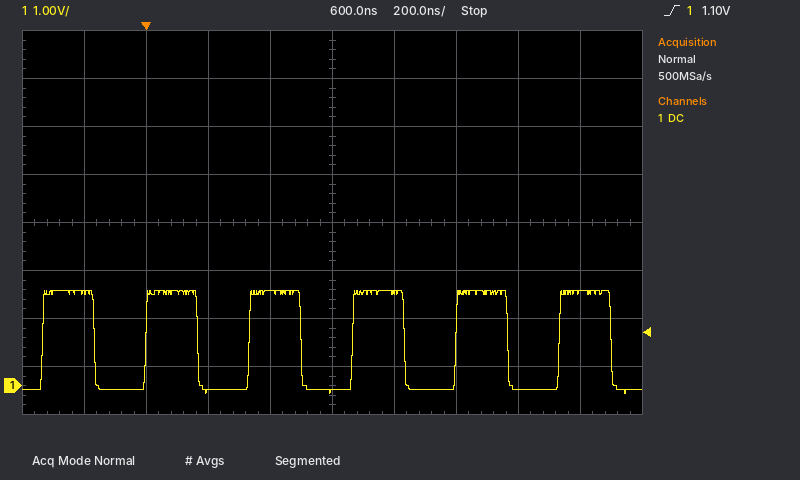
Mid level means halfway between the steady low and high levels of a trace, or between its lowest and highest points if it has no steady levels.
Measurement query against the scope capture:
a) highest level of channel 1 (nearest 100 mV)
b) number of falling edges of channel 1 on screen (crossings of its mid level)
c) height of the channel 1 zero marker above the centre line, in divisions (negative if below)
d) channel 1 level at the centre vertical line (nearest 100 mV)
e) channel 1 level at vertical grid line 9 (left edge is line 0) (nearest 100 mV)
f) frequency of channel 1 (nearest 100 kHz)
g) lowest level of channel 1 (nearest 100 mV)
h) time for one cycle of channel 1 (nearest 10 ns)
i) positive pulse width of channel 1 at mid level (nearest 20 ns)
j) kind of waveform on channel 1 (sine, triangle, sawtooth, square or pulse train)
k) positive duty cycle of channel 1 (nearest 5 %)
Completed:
2.0 V
6
-3.4 div
-100 mV
1.9 V
3.0 MHz
-200 mV
330 ns
160 ns
square
50 %
